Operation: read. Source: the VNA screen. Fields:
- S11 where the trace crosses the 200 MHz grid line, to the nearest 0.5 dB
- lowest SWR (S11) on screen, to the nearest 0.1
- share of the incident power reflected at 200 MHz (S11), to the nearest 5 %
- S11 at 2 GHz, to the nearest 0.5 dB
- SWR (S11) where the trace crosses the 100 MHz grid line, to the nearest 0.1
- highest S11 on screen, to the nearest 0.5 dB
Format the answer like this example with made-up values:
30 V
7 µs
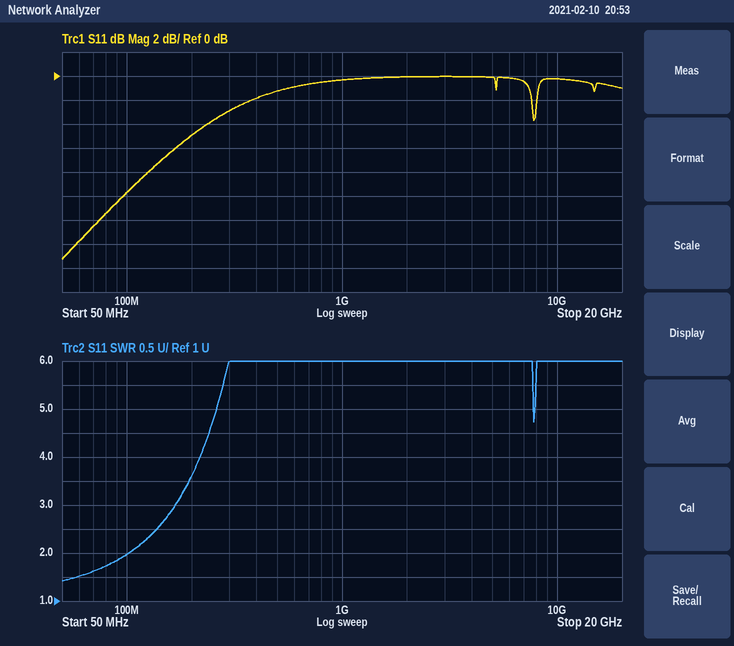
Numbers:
-5.0 dB
1.4
30 %
0.0 dB
2.0
0.0 dB
